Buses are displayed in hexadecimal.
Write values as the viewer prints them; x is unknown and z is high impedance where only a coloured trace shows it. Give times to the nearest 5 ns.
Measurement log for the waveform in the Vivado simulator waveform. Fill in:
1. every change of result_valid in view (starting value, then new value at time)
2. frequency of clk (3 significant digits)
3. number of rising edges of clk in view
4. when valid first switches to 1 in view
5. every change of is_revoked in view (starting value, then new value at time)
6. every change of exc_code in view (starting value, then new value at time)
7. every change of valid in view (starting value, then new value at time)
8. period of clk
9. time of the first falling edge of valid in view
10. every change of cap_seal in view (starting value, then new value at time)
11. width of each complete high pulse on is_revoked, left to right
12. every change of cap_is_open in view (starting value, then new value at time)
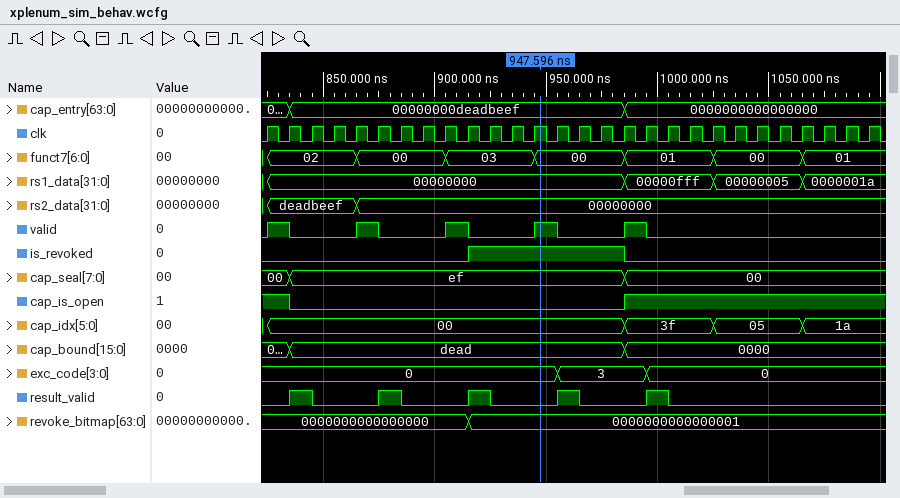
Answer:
0, 1 at 835 ns, 0 at 845 ns, 1 at 875 ns, 0 at 885 ns, 1 at 915 ns, 0 at 925 ns, 1 at 955 ns, 0 at 965 ns, 1 at 995 ns, 0 at 1005 ns
100 MHz
28
825 ns
0, 1 at 915 ns, 0 at 985 ns
0, 3 at 955 ns, 0 at 995 ns
0, 1 at 825 ns, 0 at 835 ns, 1 at 865 ns, 0 at 875 ns, 1 at 905 ns, 0 at 915 ns, 1 at 945 ns, 0 at 955 ns, 1 at 985 ns, 0 at 995 ns
10 ns
835 ns
00, ef at 835 ns, 00 at 985 ns
70 ns
1, 0 at 835 ns, 1 at 985 ns
